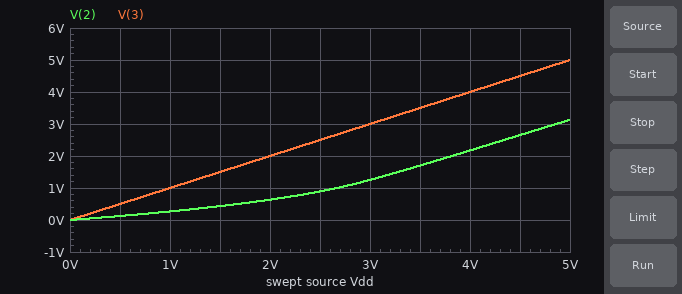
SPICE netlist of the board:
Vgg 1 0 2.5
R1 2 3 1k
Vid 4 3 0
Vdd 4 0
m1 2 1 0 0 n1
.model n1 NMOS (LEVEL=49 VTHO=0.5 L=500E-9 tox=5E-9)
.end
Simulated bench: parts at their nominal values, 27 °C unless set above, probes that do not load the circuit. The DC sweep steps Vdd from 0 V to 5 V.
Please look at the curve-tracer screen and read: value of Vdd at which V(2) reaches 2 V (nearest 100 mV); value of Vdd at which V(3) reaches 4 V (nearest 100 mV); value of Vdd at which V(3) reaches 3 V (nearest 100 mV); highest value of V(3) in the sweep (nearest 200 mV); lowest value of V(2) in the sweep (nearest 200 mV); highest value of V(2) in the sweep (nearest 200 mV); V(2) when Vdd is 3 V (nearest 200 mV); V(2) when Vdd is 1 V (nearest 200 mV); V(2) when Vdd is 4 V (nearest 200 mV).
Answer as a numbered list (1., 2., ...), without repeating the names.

1. 3.8 V
2. 4.0 V
3. 3.0 V
4. 5.0 V
5. 0 V
6. 3.2 V
7. 1.2 V
8. 200 mV
9. 2.2 V
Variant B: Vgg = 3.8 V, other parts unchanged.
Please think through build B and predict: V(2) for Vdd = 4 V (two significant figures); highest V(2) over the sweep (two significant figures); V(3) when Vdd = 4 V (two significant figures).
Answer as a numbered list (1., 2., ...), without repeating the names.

1. 1.1 V
2. 1.6 V
3. 4.0 V
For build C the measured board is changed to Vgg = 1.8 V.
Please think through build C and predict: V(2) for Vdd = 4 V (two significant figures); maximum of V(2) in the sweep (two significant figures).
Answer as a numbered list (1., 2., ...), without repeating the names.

1. 3.0 V
2. 3.9 V
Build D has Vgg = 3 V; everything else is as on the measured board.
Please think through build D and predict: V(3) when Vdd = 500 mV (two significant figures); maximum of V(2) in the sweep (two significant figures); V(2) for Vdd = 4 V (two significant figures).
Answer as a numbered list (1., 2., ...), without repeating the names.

1. 500 mV
2. 2.5 V
3. 1.6 V
